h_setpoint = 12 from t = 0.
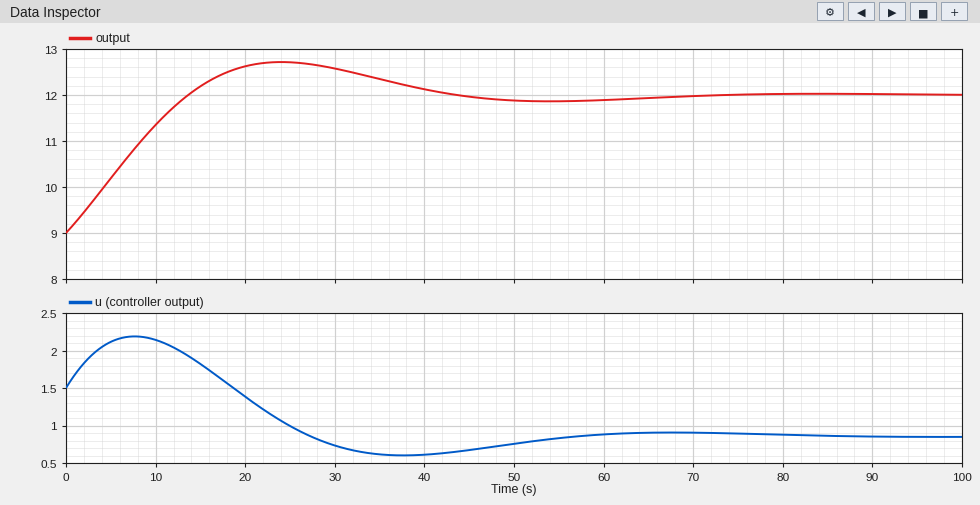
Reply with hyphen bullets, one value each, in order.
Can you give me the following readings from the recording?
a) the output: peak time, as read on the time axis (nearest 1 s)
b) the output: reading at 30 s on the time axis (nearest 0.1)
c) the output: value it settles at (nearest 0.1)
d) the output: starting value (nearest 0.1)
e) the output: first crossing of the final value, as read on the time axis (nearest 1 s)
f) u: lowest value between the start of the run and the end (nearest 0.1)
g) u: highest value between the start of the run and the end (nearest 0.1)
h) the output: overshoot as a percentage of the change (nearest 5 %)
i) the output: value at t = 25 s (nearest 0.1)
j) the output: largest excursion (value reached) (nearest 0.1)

- 24 s
- 12.6
- 12.0
- 9.0
- 14 s
- 0.6
- 2.2
- 25 %
- 12.7
- 12.7
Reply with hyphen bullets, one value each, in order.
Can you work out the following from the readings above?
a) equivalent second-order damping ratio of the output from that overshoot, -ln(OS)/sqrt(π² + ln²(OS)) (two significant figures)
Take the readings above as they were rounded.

- 0.40
